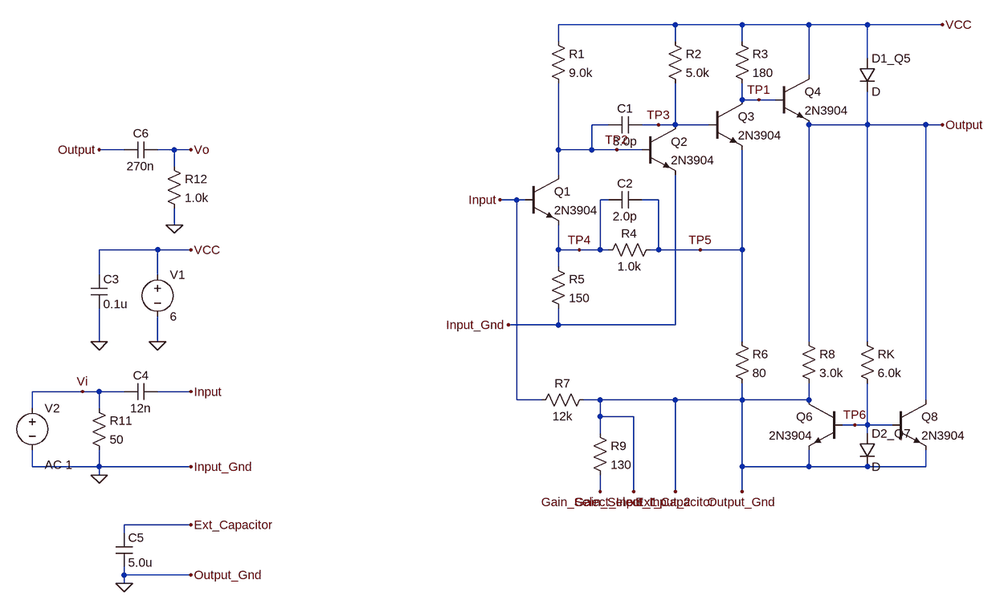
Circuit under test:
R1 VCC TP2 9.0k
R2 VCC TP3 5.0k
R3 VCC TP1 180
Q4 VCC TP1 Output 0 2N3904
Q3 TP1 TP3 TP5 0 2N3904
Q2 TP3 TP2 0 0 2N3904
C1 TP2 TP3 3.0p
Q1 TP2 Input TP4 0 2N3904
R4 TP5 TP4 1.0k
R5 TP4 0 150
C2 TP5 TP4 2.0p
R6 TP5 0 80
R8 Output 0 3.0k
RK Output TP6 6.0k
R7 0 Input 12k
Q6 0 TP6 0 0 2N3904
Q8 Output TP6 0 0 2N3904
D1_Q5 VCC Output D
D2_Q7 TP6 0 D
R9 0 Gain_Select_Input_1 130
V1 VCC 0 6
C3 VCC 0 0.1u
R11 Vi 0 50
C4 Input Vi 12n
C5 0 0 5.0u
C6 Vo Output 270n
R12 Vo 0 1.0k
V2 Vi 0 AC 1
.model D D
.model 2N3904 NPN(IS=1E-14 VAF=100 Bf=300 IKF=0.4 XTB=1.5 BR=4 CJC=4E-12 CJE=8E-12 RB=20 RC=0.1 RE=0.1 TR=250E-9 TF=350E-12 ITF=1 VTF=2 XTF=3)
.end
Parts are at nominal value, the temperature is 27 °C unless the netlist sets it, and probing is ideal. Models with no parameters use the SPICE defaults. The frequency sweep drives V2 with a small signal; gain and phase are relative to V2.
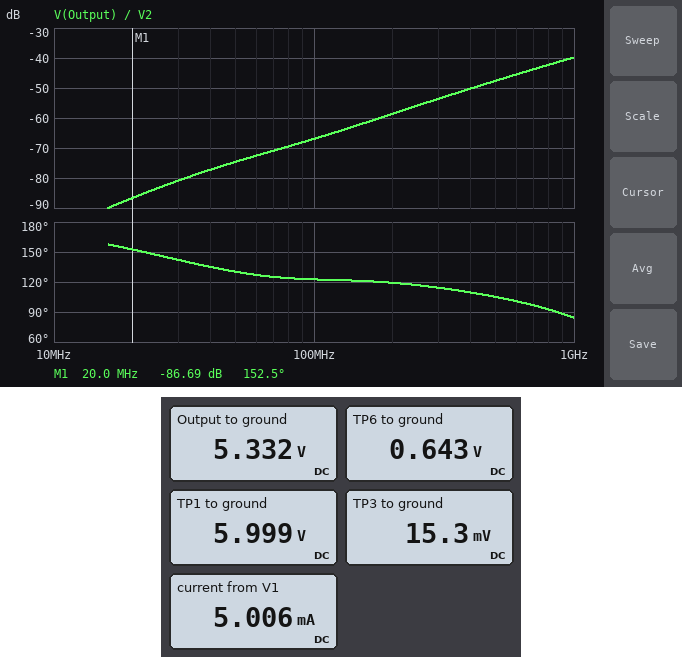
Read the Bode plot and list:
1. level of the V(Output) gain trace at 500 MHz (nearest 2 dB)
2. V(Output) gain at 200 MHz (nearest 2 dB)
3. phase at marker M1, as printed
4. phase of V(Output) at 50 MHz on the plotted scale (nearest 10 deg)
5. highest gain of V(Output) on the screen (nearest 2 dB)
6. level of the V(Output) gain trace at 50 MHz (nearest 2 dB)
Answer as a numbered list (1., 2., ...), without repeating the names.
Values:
1. -48 dB
2. -58 dB
3. 152.5 deg
4. 130 deg
5. -40 dB
6. -74 dB
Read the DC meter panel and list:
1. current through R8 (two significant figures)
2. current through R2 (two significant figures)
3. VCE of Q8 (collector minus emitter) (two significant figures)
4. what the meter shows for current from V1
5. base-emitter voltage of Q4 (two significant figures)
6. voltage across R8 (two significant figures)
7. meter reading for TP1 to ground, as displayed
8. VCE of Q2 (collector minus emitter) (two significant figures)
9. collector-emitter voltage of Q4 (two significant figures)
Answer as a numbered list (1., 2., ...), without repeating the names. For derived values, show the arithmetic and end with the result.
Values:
1. (5.332 V) / 3 kΩ = 1.8 mA
2. (6 V - 15.3 mV) / 5 kΩ = 1.2 mA
3. 5.332 V = 5.3 V
4. 5.006 mA
5. 5.999 V - 5.332 V = 670 mV
6. 5.332 V = 5.3 V
7. 5.999 V
8. 15.3 mV = 15 mV
9. 6 V - 5.332 V = 670 mV
